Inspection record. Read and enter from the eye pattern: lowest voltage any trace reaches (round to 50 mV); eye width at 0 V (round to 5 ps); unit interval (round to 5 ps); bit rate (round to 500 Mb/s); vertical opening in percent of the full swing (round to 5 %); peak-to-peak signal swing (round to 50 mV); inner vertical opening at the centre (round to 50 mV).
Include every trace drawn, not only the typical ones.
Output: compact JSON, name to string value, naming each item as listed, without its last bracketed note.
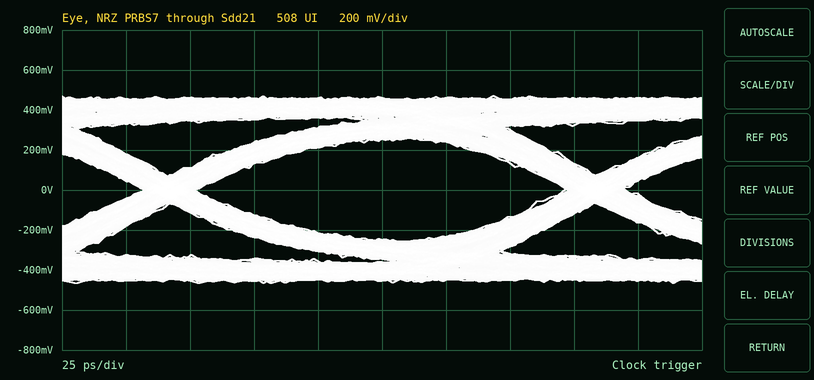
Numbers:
{"lowest voltage any trace reaches": "-450 mV", "eye width at 0 V": "145 ps", "unit interval": "165 ps", "bit rate": "6.0 Gb/s", "vertical opening in percent of the full swing": "55 %", "peak-to-peak signal swing": "950 mV", "inner vertical opening at the centre": "500 mV"}
